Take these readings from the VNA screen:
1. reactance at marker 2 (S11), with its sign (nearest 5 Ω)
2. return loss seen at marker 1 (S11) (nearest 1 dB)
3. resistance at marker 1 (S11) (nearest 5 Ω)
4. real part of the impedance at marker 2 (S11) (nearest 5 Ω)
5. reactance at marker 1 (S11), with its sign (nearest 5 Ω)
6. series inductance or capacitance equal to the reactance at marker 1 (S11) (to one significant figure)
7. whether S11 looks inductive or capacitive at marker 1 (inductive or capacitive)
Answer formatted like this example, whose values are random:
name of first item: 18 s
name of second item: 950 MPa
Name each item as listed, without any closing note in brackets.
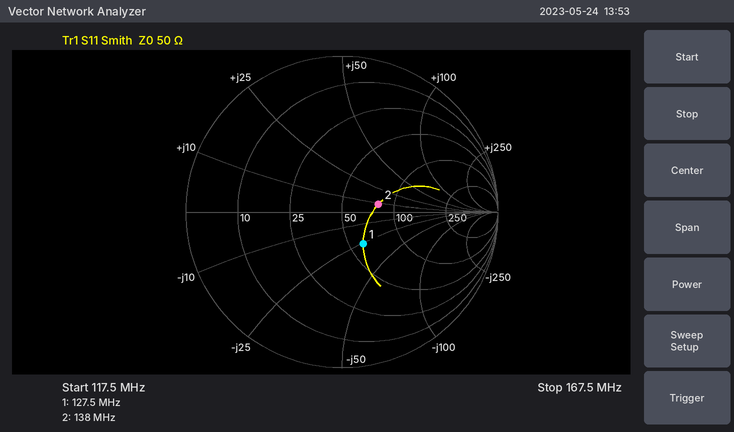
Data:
reactance at marker 2 (S11), with its sign: +10 Ω
return loss seen at marker 1 (S11): 12 dB
resistance at marker 1 (S11): 60 Ω
real part of the impedance at marker 2 (S11): 80 Ω
reactance at marker 1 (S11), with its sign: -25 Ω
series inductance or capacitance equal to the reactance at marker 1 (S11): 50 pF
whether S11 looks inductive or capacitive at marker 1: capacitive
